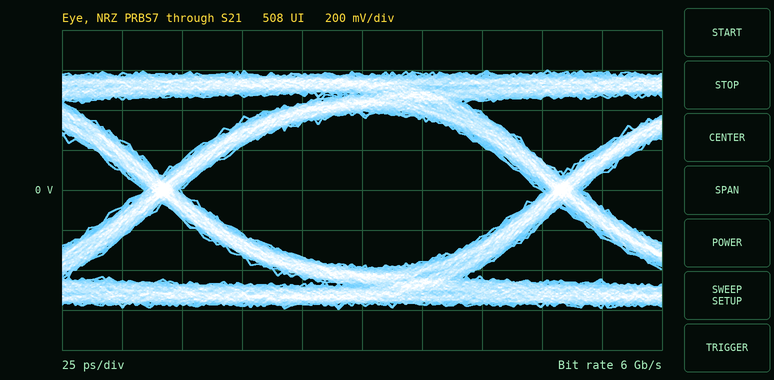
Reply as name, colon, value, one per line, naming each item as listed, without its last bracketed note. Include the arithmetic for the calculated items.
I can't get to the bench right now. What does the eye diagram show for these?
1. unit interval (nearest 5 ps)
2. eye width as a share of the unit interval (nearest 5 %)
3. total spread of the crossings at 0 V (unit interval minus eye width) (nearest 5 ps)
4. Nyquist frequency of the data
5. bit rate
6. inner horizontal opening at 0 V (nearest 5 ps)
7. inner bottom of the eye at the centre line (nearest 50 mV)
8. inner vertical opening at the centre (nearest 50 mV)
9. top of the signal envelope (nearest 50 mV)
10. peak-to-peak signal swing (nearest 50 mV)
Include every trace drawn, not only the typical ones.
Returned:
unit interval: 165 ps
eye width as a share of the unit interval: 150 ps / 165 ps ≈ 90.9 %, so 90 % to the nearest 5 %
total spread of the crossings at 0 V (unit interval minus eye width): 15 ps
Nyquist frequency of the data: 3 GHz
bit rate: 6 Gb/s
inner horizontal opening at 0 V: 150 ps
inner bottom of the eye at the centre line: -400 mV
inner vertical opening at the centre: 750 mV
top of the signal envelope: 600 mV
peak-to-peak signal swing: 1.20 V
